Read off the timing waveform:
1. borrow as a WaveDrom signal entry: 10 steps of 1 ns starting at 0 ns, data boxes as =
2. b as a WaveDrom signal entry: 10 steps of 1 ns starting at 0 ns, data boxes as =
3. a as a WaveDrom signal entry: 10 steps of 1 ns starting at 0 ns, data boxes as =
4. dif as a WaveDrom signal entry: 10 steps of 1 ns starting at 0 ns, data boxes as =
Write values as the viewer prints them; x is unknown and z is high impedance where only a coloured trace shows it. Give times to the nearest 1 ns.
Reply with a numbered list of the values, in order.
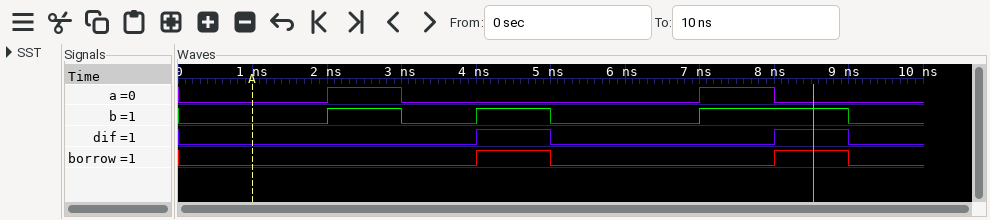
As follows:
1. {name: 'borrow', wave: '0...10..10'}
2. {name: 'b', wave: '0.1010.1.0'}
3. {name: 'a', wave: '0.10...10.'}
4. {name: 'dif', wave: '0...10..10'}
